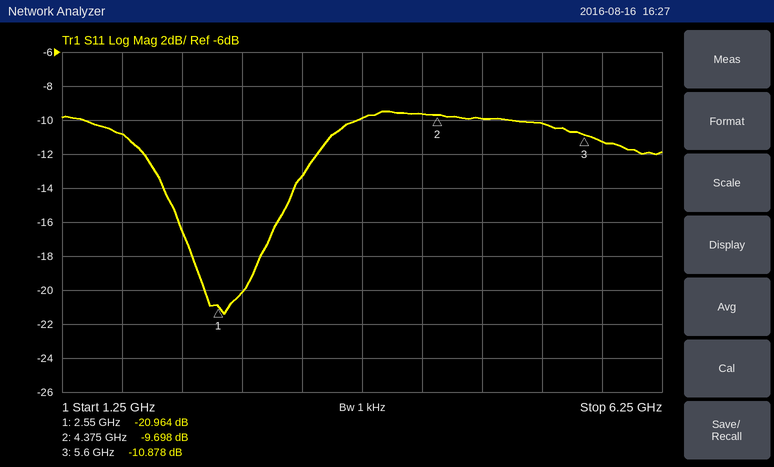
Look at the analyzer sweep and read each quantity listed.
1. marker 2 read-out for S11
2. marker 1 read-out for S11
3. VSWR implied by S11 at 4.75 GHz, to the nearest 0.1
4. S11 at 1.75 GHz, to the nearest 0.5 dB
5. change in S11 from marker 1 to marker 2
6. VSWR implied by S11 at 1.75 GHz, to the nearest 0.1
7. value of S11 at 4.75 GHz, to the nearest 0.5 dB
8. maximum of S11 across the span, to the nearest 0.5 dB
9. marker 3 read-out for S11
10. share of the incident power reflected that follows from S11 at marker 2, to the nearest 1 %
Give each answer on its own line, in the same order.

-9.698 dB
-20.964 dB
1.9
-11.0 dB
11.266 dB
1.8
-10.0 dB
-9.5 dB
-10.878 dB
11 %
